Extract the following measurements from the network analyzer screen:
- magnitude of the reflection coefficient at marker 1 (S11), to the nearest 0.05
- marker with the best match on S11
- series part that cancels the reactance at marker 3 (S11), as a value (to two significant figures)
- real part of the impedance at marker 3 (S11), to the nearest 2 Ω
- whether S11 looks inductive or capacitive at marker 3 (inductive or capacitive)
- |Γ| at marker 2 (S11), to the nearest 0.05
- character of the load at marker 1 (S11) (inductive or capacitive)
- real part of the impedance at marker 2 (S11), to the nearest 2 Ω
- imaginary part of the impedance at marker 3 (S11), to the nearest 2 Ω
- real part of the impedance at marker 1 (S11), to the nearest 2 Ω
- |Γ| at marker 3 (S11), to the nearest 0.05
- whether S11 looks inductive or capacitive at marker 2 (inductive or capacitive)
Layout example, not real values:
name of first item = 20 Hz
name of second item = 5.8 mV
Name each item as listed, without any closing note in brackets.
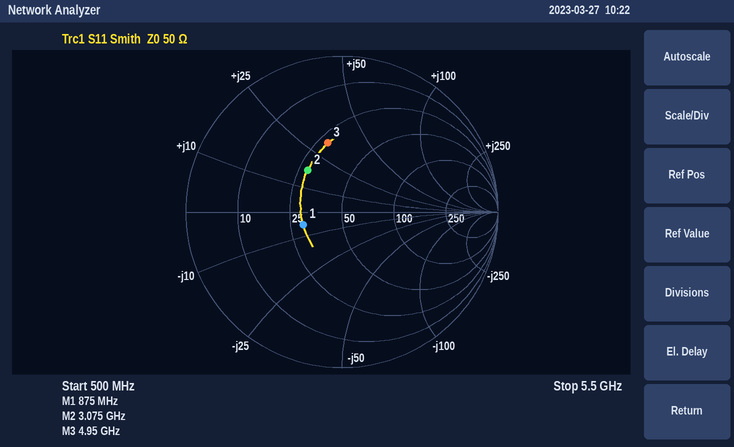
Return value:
magnitude of the reflection coefficient at marker 1 (S11), to the nearest 0.05 = 0.25
marker with the best match on S11 = marker 1
series part that cancels the reactance at marker 3 (S11), as a value = 1.0 pF
real part of the impedance at marker 3 (S11), to the nearest 2 Ω = 28 Ω
whether S11 looks inductive or capacitive at marker 3 = inductive
|Γ| at marker 2 (S11), to the nearest 0.05 = 0.35
character of the load at marker 1 (S11) = capacitive
real part of the impedance at marker 2 (S11), to the nearest 2 Ω = 28 Ω
imaginary part of the impedance at marker 3 (S11), to the nearest 2 Ω = +32 Ω
real part of the impedance at marker 1 (S11), to the nearest 2 Ω = 30 Ω
|Γ| at marker 3 (S11), to the nearest 0.05 = 0.45
whether S11 looks inductive or capacitive at marker 2 = inductive
